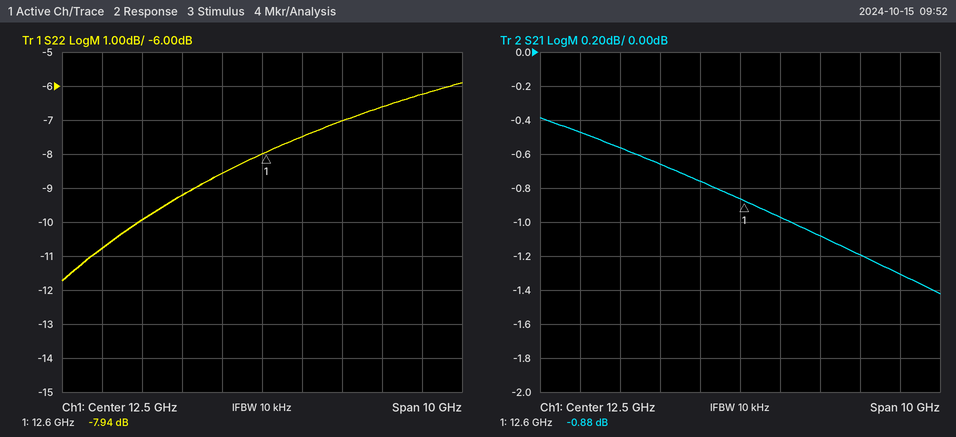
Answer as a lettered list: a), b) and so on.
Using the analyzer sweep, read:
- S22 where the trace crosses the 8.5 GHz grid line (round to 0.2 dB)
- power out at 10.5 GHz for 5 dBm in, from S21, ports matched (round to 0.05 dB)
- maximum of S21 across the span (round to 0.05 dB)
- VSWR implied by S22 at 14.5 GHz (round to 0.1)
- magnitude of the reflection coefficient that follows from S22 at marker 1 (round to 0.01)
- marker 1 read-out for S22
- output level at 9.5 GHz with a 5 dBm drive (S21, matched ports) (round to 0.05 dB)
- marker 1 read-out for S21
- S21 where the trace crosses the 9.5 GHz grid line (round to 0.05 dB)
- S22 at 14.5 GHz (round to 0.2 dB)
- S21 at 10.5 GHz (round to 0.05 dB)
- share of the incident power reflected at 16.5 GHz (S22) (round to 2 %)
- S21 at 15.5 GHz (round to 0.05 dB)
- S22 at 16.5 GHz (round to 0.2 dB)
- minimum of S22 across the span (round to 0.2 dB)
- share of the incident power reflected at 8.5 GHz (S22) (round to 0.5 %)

a) -10.8 dB
b) 4.35 dBm
c) -0.40 dB
d) 2.6
e) 0.40
f) -7.94 dB
g) 4.45 dBm
h) -0.88 dB
i) -0.55 dB
j) -7.0 dB
k) -0.65 dB
l) 24 %
m) -1.20 dB
n) -6.2 dB
o) -11.8 dB
p) 8.5 %
